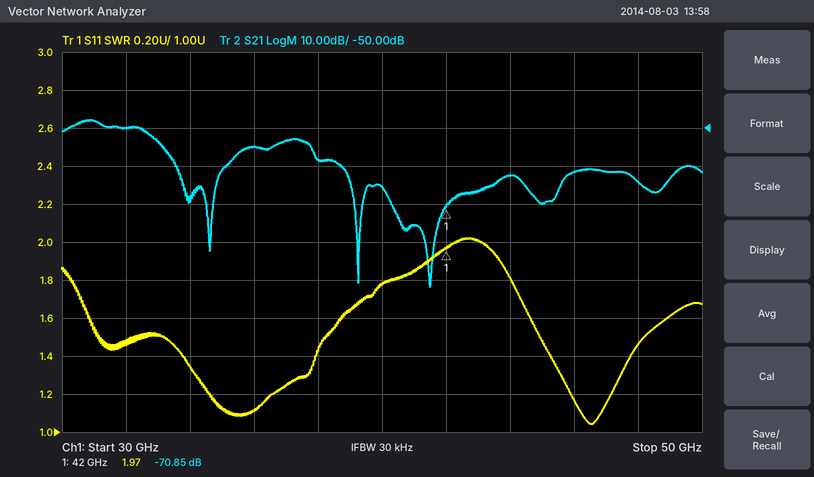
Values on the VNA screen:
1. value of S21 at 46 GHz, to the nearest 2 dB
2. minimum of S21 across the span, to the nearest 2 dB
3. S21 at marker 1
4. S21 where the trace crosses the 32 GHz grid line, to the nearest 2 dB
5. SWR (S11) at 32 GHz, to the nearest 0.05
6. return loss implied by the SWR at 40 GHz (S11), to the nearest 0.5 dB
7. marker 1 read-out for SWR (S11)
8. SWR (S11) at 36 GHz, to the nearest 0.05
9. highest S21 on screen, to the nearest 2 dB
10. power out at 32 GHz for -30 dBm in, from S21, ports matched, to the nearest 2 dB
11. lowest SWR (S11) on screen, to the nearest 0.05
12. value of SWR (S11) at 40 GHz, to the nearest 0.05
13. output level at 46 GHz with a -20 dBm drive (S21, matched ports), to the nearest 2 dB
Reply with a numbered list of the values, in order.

1. -62 dB
2. -92 dB
3. -70.85 dB
4. -50 dB
5. 1.45
6. 11.0 dB
7. 1.97
8. 1.10
9. -48 dB
10. -80 dBm
11. 1.05
12. 1.80
13. -82 dBm
